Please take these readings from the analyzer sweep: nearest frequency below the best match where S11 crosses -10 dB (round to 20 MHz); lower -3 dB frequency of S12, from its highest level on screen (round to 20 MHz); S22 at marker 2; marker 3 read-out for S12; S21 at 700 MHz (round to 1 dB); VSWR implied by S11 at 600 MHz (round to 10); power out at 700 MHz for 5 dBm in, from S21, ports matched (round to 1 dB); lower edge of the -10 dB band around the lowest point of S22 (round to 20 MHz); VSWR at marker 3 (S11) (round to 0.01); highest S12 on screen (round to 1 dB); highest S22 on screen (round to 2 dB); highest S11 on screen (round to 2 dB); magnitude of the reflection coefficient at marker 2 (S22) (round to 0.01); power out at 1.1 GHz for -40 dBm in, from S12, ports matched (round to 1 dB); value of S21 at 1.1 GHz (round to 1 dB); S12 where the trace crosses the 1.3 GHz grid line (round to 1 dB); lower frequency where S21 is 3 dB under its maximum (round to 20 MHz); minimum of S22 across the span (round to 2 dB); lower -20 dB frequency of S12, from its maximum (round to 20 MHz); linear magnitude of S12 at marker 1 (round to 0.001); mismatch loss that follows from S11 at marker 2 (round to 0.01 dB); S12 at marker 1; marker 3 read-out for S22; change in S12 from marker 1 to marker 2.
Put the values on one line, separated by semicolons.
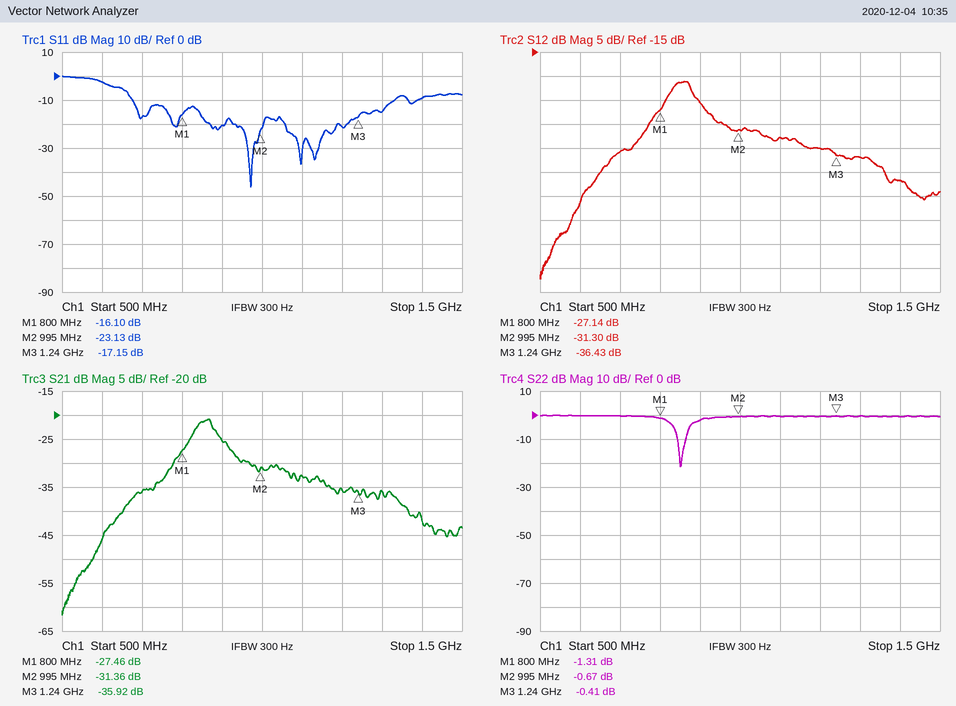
680 MHz; 820 MHz; -0.67 dB; -36.43 dB; -36 dB; 10; -31 dBm; 840 MHz; 1.32; -21 dB; 0 dB; 0 dB; 0.93; -73 dBm; -33 dB; -37 dB; 820 MHz; -22 dB; 640 MHz; 0.044; 0.02 dB; -27.14 dB; -0.41 dB; -4.16 dB
